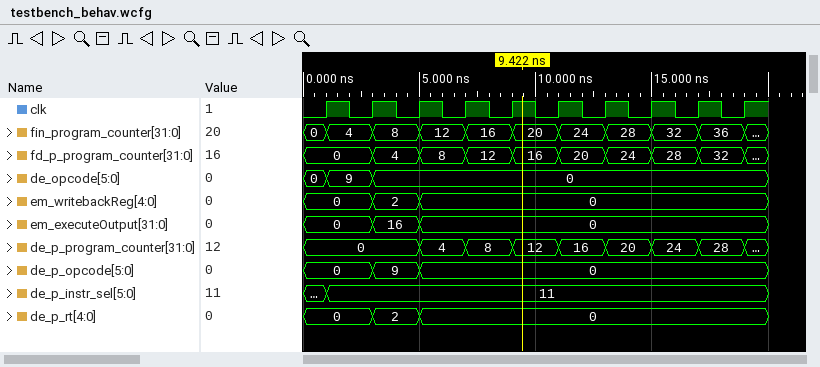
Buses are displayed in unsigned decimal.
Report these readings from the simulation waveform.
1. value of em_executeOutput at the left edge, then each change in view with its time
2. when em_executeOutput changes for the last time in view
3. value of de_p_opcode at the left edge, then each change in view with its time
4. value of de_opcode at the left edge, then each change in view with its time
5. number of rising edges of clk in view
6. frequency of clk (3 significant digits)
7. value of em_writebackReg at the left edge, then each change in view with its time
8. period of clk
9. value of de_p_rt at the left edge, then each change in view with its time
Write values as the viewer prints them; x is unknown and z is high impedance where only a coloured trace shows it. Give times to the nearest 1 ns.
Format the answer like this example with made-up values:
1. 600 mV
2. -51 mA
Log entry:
1. 0, 16 at 3 ns, 0 at 5 ns
2. 5 ns
3. 0, 9 at 3 ns, 0 at 5 ns
4. 0, 9 at 1 ns, 0 at 3 ns
5. 10
6. 500 MHz
7. 0, 2 at 3 ns, 0 at 5 ns
8. 2 ns
9. 0, 2 at 3 ns, 0 at 5 ns
